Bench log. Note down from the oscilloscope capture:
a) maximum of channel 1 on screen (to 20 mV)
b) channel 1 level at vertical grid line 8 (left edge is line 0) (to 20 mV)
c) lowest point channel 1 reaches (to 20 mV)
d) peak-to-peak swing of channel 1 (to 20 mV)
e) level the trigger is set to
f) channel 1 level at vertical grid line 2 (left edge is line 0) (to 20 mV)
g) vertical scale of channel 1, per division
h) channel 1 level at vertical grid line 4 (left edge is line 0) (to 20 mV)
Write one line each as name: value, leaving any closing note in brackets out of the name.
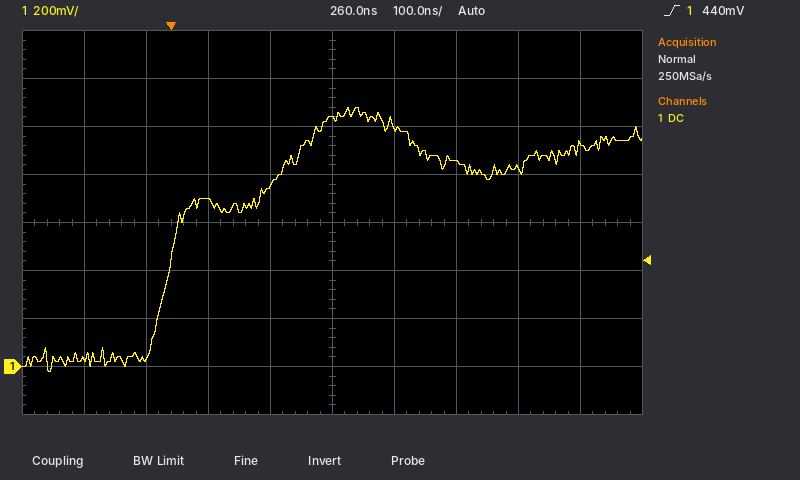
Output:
maximum of channel 1 on screen: 1.08 V
channel 1 level at vertical grid line 8 (left edge is line 0): 820 mV
lowest point channel 1 reaches: -20 mV
peak-to-peak swing of channel 1: 1.10 V
level the trigger is set to: 440 mV
channel 1 level at vertical grid line 2 (left edge is line 0): 40 mV
vertical scale of channel 1, per division: 200 mV
channel 1 level at vertical grid line 4 (left edge is line 0): 760 mV
